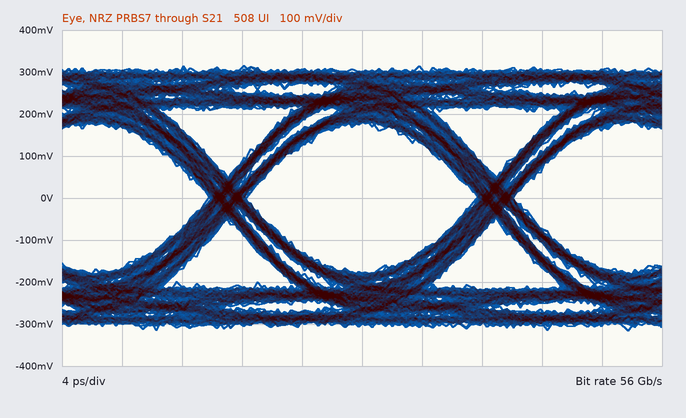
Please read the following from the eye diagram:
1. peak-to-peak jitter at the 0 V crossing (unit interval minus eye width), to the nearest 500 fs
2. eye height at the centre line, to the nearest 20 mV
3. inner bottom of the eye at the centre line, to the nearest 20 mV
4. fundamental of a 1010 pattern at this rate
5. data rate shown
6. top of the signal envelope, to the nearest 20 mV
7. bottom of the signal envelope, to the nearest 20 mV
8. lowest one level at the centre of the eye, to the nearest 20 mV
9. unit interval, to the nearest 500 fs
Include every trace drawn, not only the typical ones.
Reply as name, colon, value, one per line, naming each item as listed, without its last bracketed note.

peak-to-peak jitter at the 0 V crossing (unit interval minus eye width), to the nearest 500 fs: 2.5 ps
eye height at the centre line, to the nearest 20 mV: 360 mV
inner bottom of the eye at the centre line, to the nearest 20 mV: -180 mV
fundamental of a 1010 pattern at this rate: 28 GHz
data rate shown: 56 Gb/s
top of the signal envelope, to the nearest 20 mV: 320 mV
bottom of the signal envelope, to the nearest 20 mV: -320 mV
lowest one level at the centre of the eye, to the nearest 20 mV: 180 mV
unit interval, to the nearest 500 fs: 18.0 ps
